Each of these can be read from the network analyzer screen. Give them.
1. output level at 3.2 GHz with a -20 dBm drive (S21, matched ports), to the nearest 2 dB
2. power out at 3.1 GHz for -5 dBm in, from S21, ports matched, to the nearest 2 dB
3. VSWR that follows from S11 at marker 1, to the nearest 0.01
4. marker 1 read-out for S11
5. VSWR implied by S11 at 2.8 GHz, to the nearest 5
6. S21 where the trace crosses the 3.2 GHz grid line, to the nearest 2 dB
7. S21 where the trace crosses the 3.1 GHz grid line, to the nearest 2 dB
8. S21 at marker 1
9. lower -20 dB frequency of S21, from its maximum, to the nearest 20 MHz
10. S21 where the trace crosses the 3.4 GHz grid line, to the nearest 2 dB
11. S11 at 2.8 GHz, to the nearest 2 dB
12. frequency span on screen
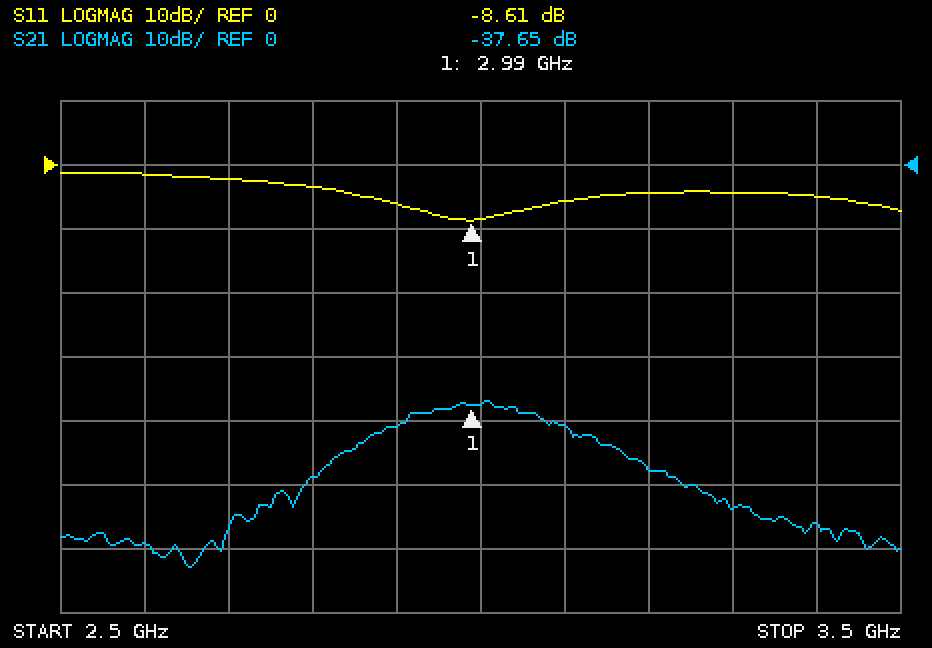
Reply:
-68 dBm
-46 dBm
2.18
-8.61 dB
5
-48 dB
-40 dB
-37.65 dB
2.70 GHz
-56 dB
-4 dB
1 GHz
